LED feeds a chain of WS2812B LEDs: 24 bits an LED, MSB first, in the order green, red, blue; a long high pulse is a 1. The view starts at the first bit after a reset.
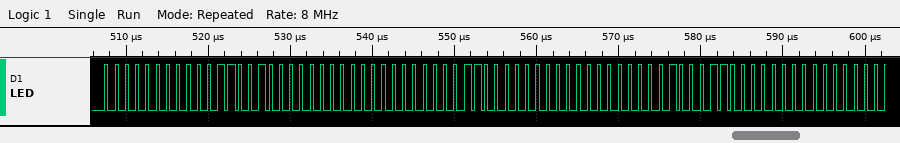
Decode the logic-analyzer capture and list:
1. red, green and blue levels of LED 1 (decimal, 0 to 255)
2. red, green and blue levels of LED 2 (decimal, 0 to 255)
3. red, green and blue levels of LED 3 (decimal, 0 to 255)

25, 0, 0
24, 0, 0
24, 1, 0
